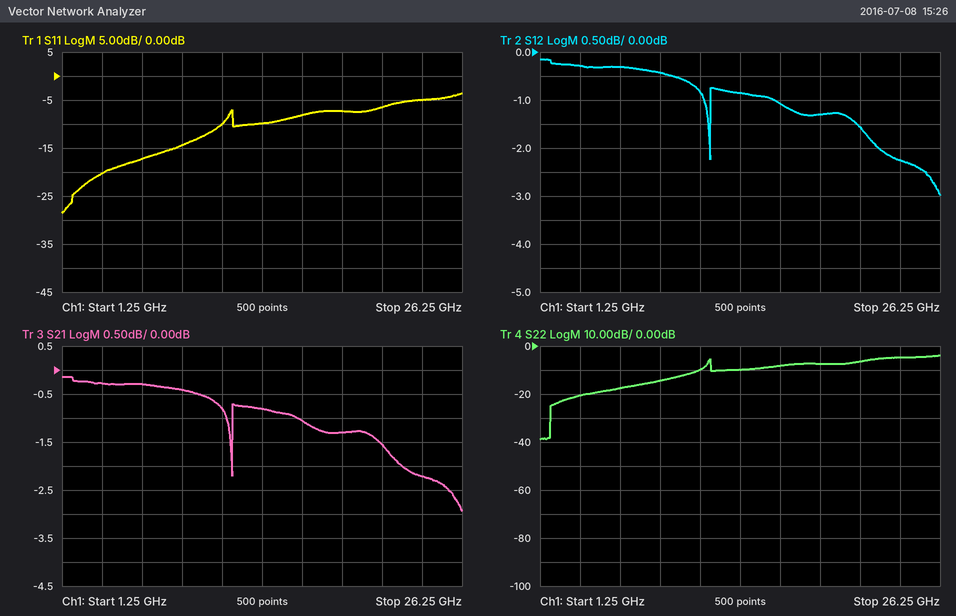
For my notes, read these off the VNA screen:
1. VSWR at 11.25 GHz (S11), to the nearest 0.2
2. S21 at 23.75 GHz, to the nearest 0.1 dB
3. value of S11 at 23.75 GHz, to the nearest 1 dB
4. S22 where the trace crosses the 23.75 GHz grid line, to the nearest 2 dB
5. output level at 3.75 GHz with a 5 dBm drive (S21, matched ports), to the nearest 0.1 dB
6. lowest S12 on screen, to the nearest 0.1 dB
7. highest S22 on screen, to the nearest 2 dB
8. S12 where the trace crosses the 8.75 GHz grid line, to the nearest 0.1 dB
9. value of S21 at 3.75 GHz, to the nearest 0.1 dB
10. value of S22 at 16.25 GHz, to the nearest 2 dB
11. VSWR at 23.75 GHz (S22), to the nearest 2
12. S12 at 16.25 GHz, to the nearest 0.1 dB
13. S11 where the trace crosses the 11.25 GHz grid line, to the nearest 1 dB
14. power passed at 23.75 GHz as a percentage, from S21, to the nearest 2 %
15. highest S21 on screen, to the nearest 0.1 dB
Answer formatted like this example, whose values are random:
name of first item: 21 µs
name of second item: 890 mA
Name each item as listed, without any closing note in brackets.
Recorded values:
VSWR at 11.25 GHz (S11), to the nearest 0.2: 2.0
S21 at 23.75 GHz, to the nearest 0.1 dB: -2.2 dB
value of S11 at 23.75 GHz, to the nearest 1 dB: -5 dB
S22 where the trace crosses the 23.75 GHz grid line, to the nearest 2 dB: -4 dB
output level at 3.75 GHz with a 5 dBm drive (S21, matched ports), to the nearest 0.1 dB: 4.7 dBm
lowest S12 on screen, to the nearest 0.1 dB: -3.0 dB
highest S22 on screen, to the nearest 2 dB: -4 dB
S12 where the trace crosses the 8.75 GHz grid line, to the nearest 0.1 dB: -0.4 dB
value of S21 at 3.75 GHz, to the nearest 0.1 dB: -0.3 dB
value of S22 at 16.25 GHz, to the nearest 2 dB: -8 dB
VSWR at 23.75 GHz (S22), to the nearest 2: 4
S12 at 16.25 GHz, to the nearest 0.1 dB: -1.1 dB
S11 where the trace crosses the 11.25 GHz grid line, to the nearest 1 dB: -10 dB
power passed at 23.75 GHz as a percentage, from S21, to the nearest 2 %: 60 %
highest S21 on screen, to the nearest 0.1 dB: -0.1 dB
